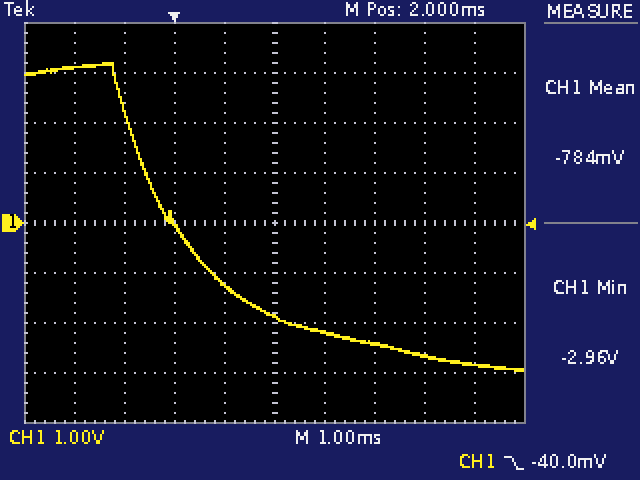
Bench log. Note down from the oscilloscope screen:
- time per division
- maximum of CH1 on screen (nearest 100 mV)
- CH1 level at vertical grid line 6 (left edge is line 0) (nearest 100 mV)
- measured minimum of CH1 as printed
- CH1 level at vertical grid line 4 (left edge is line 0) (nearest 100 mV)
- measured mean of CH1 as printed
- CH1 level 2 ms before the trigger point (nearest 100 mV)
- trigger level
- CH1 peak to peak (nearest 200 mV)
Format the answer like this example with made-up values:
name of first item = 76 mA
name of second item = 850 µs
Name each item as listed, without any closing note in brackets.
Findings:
time per division = 1 ms
maximum of CH1 on screen = 3.2 V
CH1 level at vertical grid line 6 (left edge is line 0) = -2.2 V
measured minimum of CH1 as printed = -2.96 V
CH1 level at vertical grid line 4 (left edge is line 0) = -1.2 V
measured mean of CH1 as printed = -784 mV
CH1 level 2 ms before the trigger point = 3.1 V
trigger level = -40.0 mV
CH1 peak to peak = 6.2 V
